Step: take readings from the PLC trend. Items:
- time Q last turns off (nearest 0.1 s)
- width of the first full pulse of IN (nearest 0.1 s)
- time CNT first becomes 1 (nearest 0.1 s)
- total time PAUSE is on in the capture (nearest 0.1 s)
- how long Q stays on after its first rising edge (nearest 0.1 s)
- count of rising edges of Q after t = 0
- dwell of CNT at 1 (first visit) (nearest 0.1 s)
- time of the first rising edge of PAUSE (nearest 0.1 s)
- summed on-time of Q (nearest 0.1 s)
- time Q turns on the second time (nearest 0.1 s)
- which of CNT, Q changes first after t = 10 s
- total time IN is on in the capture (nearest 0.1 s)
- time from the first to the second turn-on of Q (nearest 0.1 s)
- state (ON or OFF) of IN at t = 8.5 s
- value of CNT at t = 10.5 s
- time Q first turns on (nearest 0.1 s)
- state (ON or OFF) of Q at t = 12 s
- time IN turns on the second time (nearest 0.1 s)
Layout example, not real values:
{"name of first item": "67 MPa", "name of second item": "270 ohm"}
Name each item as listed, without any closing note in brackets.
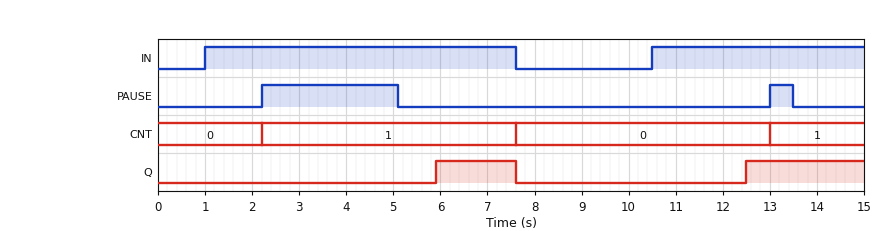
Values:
{"time Q last turns off": "7.6 s", "width of the first full pulse of IN": "6.6 s", "time CNT first becomes 1": "2.2 s", "total time PAUSE is on in the capture": "3.4 s", "how long Q stays on after its first rising edge": "1.7 s", "count of rising edges of Q after t = 0": "2", "dwell of CNT at 1 (first visit)": "5.4 s", "time of the first rising edge of PAUSE": "2.2 s", "summed on-time of Q": "4.2 s", "time Q turns on the second time": "12.5 s", "which of CNT, Q changes first after t = 10 s": "Q", "total time IN is on in the capture": "11.1 s", "time from the first to the second turn-on of Q": "6.6 s", "state (ON or OFF) of IN at t = 8.5 s": "OFF", "value of CNT at t = 10.5 s": "0", "time Q first turns on": "5.9 s", "state (ON or OFF) of Q at t = 12 s": "OFF", "time IN turns on the second time": "10.5 s"}
